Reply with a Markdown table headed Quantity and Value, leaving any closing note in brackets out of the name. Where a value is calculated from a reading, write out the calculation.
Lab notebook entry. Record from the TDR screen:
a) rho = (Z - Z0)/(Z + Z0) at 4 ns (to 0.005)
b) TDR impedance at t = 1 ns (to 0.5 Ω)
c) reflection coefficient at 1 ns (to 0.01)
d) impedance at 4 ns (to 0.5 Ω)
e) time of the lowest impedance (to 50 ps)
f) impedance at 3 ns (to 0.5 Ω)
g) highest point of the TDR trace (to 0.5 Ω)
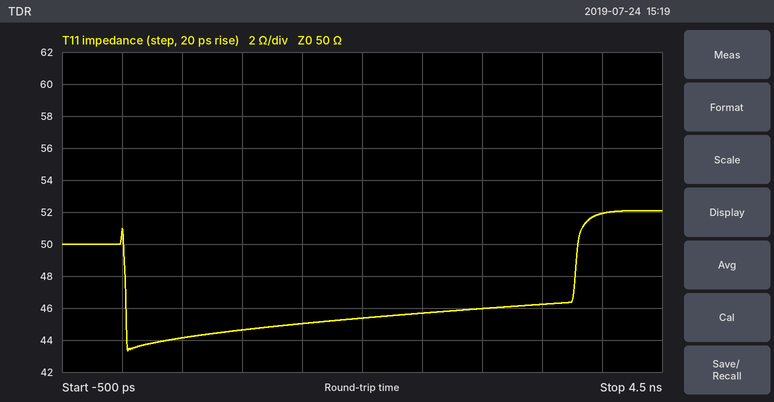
| Quantity | Value |
|---|---|
| rho = (Z - Z0)/(Z + Z0) at 4 ns | (52 − 50)/(52 + 50) ≈ +0.020 |
| TDR impedance at t = 1 ns | 44.5 Ω |
| reflection coefficient at 1 ns | (44.5 − 50)/(44.5 + 50) ≈ -0.06 |
| impedance at 4 ns | 52.0 Ω |
| time of the lowest impedance | 50 ps |
| impedance at 3 ns | 46.0 Ω |
| highest point of the TDR trace | 52.0 Ω |
